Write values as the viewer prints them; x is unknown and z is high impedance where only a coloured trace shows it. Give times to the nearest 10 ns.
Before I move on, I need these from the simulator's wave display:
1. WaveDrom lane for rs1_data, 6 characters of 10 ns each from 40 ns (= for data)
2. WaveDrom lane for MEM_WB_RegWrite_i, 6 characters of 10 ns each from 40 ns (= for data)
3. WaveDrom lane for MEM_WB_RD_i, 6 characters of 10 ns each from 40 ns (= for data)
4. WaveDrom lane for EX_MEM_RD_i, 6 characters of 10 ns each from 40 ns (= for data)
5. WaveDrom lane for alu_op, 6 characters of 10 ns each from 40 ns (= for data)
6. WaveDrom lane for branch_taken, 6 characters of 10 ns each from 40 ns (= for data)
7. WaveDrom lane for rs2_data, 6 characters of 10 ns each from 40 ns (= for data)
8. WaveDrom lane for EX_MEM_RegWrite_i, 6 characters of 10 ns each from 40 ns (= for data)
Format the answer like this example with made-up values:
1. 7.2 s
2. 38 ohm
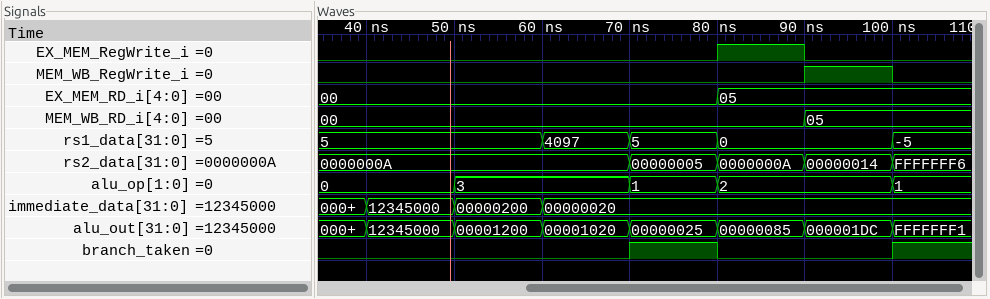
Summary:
1. {name: 'rs1_data', wave: '=.===.', data: '5 4097 5 0'}
2. {name: 'MEM_WB_RegWrite_i', wave: '0....1'}
3. {name: 'MEM_WB_RD_i', wave: '=....=', data: '00 05'}
4. {name: 'EX_MEM_RD_i', wave: '=...=.', data: '00 05'}
5. {name: 'alu_op', wave: '==.==.', data: '0 3 1 2'}
6. {name: 'branch_taken', wave: '0..10.'}
7. {name: 'rs2_data', wave: '=..===', data: '0000000A 00000005 0000000A 00000014'}
8. {name: 'EX_MEM_RegWrite_i', wave: '0...10'}
